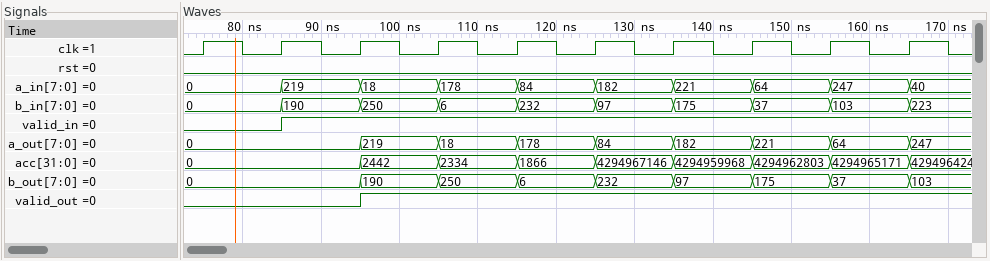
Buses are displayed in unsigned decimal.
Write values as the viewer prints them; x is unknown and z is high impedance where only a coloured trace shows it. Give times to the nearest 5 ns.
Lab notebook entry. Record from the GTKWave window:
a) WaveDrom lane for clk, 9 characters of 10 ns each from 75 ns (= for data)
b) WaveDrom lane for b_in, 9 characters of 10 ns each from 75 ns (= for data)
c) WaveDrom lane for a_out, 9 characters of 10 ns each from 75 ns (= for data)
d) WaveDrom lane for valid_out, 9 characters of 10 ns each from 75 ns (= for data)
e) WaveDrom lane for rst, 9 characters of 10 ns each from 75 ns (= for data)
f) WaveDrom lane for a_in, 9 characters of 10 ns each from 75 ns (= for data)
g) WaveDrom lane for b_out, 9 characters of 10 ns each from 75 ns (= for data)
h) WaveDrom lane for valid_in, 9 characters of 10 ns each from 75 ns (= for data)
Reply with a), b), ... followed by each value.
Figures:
a) {name: 'clk', wave: 'p........'}
b) {name: 'b_in', wave: '=========', data: '0 190 250 6 232 97 175 37 103'}
c) {name: 'a_out', wave: '=.=======', data: '0 219 18 178 84 182 221 64'}
d) {name: 'valid_out', wave: '0.1......'}
e) {name: 'rst', wave: '0........'}
f) {name: 'a_in', wave: '=========', data: '0 219 18 178 84 182 221 64 247'}
g) {name: 'b_out', wave: '=.=======', data: '0 190 250 6 232 97 175 37'}
h) {name: 'valid_in', wave: '01.......'}
